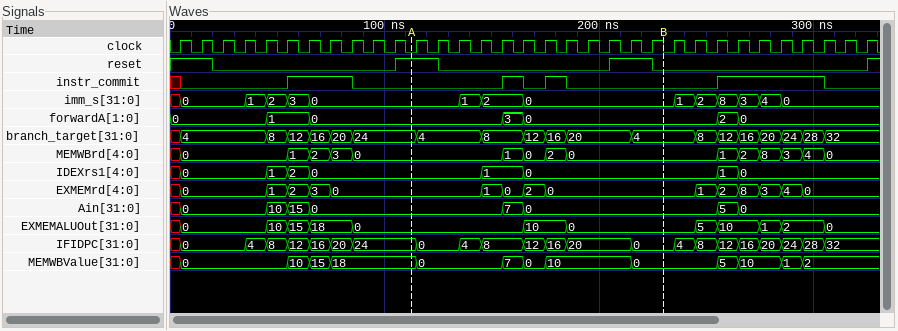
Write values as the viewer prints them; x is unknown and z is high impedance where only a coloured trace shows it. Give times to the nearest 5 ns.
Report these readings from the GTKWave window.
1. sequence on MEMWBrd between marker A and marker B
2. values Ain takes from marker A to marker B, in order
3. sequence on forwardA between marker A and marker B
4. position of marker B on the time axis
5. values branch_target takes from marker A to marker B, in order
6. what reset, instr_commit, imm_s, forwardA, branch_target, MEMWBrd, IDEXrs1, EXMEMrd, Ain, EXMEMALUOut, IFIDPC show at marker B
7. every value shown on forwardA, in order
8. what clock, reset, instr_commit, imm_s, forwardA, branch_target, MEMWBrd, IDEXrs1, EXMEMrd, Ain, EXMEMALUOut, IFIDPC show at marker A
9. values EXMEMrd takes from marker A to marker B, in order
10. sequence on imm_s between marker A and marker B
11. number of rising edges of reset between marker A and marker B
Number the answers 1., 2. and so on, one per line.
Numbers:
1. 0, 1, 0, 2, 0
2. 0, 7, 0
3. 0, 3, 0
4. 230 ns
5. 24, 4, 8, 12, 16, 20, 4
6. reset=0, instr_commit=0, imm_s=0, forwardA=0, branch_target=4, MEMWBrd=0, IDEXrs1=0, EXMEMrd=0, Ain=0, EXMEMALUOut=0, IFIDPC=0
7. 0, 1, 0, 3, 0, 2, 0
8. clock=0, reset=1, instr_commit=0, imm_s=0, forwardA=0, branch_target=24, MEMWBrd=0, IDEXrs1=0, EXMEMrd=0, Ain=0, EXMEMALUOut=0, IFIDPC=24
9. 0, 1, 0, 2, 0
10. 0, 1, 2, 0
11. 1
